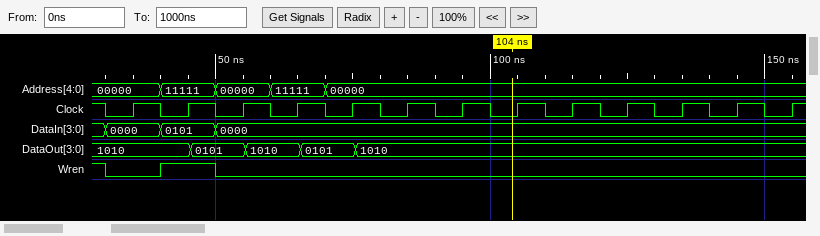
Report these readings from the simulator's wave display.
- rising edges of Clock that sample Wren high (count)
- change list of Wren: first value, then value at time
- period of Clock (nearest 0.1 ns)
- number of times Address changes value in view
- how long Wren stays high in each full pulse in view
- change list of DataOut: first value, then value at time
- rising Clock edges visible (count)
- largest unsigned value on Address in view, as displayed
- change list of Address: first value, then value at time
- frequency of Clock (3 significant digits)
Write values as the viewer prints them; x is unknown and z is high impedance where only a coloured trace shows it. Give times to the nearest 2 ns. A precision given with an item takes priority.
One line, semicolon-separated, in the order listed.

1; 1, 0 at 30 ns, 1 at 40 ns, 0 at 50 ns; 10 ns; 4; 10 ns; 1010, 0101 at 46 ns, 1010 at 56 ns, 0101 at 66 ns, 1010 at 76 ns; 13; 11111; 00000, 11111 at 40 ns, 00000 at 50 ns, 11111 at 60 ns, 00000 at 70 ns; 100 MHz
